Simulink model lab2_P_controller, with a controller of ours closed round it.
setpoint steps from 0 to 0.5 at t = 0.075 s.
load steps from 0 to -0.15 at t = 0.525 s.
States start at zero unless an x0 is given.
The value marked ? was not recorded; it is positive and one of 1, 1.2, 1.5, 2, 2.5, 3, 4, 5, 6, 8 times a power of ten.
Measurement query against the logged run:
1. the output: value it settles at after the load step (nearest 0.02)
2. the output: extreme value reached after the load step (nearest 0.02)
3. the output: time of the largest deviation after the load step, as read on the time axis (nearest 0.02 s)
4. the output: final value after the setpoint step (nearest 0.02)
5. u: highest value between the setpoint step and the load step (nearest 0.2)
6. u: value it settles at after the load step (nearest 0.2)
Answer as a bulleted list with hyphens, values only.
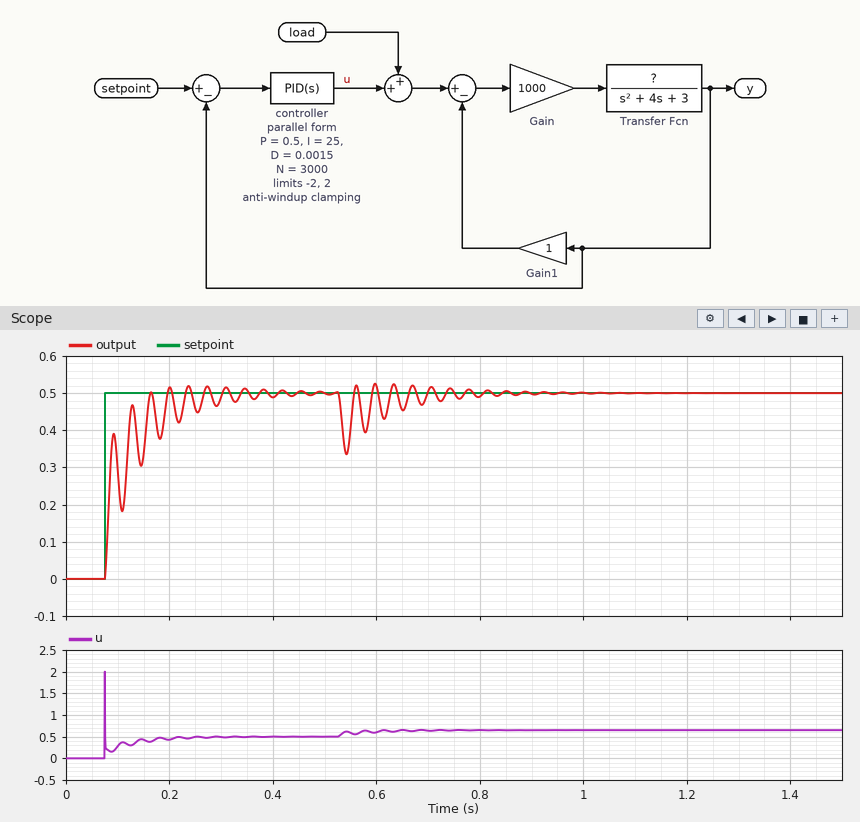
- 0.50
- 0.34
- 0.54 s
- 0.50
- 2.0
- 0.6
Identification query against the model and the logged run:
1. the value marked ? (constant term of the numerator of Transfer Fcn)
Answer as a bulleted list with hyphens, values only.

- 20
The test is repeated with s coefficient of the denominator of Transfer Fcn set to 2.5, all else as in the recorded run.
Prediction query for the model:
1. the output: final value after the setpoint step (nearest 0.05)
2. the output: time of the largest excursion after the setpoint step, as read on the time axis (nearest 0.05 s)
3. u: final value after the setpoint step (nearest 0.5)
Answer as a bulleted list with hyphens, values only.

- 0.50
- 0.25 s
- 0.5
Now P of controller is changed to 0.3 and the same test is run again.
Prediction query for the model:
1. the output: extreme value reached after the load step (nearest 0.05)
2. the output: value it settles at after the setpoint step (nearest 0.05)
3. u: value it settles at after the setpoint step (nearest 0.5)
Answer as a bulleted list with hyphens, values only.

- 0.30
- 0.50
- 0.5
